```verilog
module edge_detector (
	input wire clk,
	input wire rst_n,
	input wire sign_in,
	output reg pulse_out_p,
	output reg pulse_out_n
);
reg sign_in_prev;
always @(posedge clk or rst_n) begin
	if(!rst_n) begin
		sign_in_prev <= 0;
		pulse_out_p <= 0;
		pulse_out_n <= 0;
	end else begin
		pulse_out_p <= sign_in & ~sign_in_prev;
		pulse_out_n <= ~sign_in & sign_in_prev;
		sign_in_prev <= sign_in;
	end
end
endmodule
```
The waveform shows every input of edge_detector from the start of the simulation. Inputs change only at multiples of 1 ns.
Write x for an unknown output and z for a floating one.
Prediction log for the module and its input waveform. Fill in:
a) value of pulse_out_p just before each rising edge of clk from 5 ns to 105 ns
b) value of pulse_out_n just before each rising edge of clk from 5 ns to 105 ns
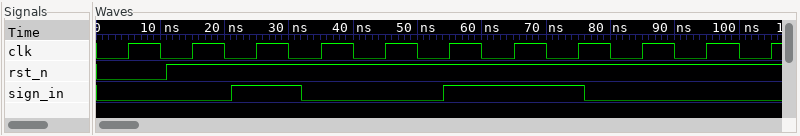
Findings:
0 0 0 1 0 0 1 0 0 0 0
0 0 0 0 1 0 0 0 0 1 0
